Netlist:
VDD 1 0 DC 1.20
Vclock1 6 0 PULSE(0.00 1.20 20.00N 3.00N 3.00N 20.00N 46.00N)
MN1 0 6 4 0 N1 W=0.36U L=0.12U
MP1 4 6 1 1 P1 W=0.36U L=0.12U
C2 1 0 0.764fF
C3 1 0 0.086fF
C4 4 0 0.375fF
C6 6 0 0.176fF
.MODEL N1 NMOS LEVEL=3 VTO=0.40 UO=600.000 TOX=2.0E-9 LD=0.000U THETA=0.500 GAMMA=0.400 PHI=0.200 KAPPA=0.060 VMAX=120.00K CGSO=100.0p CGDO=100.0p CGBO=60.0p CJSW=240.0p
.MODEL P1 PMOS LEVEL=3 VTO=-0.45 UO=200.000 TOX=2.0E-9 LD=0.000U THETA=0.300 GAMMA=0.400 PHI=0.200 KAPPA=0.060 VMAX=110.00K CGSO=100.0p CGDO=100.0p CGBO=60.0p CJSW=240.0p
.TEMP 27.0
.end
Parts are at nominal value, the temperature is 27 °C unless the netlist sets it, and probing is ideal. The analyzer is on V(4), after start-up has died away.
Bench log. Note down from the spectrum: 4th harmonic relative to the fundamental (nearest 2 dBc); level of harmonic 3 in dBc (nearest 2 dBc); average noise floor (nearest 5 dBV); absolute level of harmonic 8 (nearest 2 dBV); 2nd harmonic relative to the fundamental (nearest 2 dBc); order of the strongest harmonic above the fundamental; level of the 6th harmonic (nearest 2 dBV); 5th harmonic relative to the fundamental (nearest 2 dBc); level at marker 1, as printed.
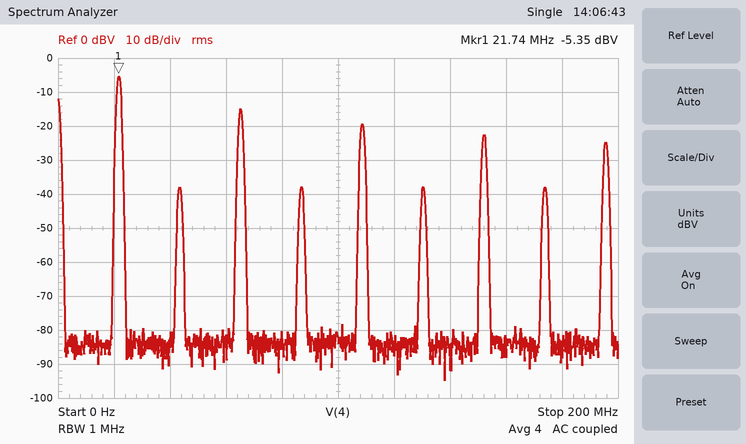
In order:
-32 dBc
-10 dBc
-85 dBV
-38 dBV
-32 dBc
3
-38 dBV
-14 dBc
-5.35 dBV
